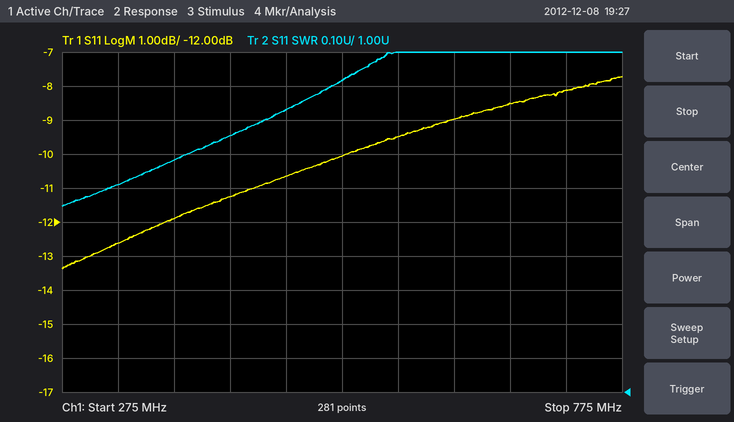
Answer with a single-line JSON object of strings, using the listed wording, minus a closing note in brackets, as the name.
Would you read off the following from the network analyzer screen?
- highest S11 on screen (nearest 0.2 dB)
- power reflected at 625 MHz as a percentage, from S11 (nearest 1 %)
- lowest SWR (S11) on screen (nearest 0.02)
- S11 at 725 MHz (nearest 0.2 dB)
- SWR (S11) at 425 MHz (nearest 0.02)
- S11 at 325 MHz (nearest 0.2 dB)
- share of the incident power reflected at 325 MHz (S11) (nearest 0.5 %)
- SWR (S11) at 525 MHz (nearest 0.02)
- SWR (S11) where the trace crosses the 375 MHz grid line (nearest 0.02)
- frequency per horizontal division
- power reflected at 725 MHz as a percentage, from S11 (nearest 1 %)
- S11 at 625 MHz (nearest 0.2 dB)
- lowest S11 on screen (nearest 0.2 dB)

{"highest S11 on screen": "-7.8 dB", "power reflected at 625 MHz as a percentage, from S11": "13 %", "lowest SWR (S11) on screen": "1.54", "S11 at 725 MHz": "-8.2 dB", "SWR (S11) at 425 MHz": "1.76", "S11 at 325 MHz": "-12.6 dB", "share of the incident power reflected at 325 MHz (S11)": "5.5 %", "SWR (S11) at 525 MHz": "1.92", "SWR (S11) where the trace crosses the 375 MHz grid line": "1.68", "frequency per horizontal division": "50 MHz", "power reflected at 725 MHz as a percentage, from S11": "15 %", "S11 at 625 MHz": "-9.0 dB", "lowest S11 on screen": "-13.4 dB"}
